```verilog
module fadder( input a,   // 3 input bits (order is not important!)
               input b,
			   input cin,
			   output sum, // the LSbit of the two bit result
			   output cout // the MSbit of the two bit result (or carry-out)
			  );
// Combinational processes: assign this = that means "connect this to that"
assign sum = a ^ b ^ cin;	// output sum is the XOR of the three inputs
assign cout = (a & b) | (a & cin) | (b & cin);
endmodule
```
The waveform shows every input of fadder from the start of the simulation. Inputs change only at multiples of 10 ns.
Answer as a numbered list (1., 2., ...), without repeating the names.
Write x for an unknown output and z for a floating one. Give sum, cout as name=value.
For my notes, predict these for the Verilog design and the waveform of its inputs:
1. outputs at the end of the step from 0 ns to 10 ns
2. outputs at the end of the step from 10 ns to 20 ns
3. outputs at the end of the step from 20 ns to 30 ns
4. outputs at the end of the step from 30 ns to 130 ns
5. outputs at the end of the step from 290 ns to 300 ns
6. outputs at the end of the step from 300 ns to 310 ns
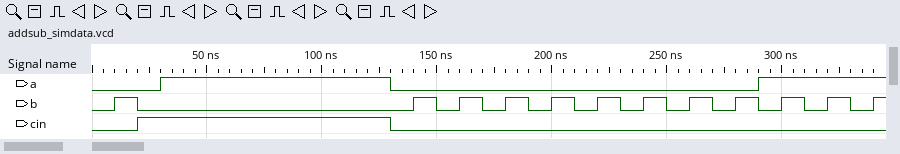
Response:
1. sum=0, cout=0
2. sum=1, cout=0
3. sum=1, cout=0
4. sum=0, cout=1
5. sum=1, cout=0
6. sum=0, cout=1
